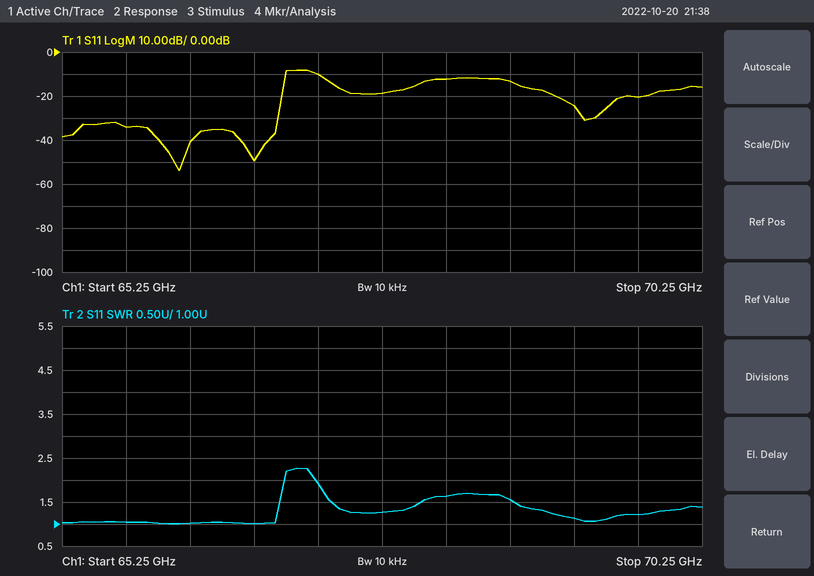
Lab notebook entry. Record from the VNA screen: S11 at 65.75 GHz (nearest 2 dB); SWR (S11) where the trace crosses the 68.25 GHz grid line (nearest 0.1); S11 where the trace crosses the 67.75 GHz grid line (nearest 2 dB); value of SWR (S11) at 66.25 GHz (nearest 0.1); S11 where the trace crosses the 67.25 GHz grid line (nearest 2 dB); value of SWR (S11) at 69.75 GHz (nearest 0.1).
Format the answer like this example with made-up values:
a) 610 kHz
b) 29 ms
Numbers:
a) -34 dB
b) 1.6
c) -18 dB
d) 1.0
e) -10 dB
f) 1.2
